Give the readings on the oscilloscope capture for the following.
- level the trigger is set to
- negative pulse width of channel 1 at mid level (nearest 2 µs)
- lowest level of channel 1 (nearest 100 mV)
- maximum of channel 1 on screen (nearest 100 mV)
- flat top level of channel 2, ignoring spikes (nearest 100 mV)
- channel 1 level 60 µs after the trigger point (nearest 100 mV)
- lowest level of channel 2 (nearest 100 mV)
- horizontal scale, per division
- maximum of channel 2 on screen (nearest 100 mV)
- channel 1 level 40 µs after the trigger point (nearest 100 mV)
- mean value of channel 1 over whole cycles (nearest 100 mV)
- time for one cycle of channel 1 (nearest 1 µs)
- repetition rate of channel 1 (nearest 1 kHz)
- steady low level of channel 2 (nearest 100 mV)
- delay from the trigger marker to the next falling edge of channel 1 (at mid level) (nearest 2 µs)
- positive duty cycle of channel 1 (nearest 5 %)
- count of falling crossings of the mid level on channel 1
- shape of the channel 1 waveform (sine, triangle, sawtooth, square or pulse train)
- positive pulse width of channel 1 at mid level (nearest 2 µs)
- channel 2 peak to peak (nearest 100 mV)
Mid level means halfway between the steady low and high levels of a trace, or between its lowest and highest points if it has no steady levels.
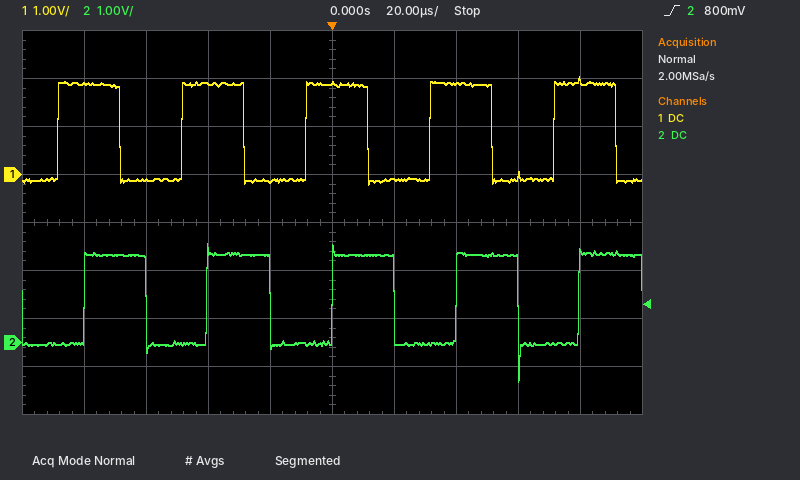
800 mV
20 µs
-200 mV
2.0 V
1.8 V
0.0 V
-800 mV
20 µs
2.1 V
1.9 V
900 mV
40 µs
25 kHz
0.0 V
12 µs
50 %
5
square
20 µs
2.9 V
